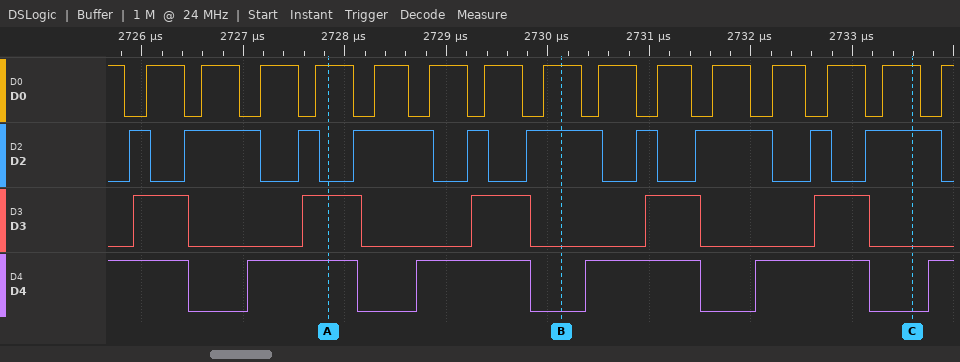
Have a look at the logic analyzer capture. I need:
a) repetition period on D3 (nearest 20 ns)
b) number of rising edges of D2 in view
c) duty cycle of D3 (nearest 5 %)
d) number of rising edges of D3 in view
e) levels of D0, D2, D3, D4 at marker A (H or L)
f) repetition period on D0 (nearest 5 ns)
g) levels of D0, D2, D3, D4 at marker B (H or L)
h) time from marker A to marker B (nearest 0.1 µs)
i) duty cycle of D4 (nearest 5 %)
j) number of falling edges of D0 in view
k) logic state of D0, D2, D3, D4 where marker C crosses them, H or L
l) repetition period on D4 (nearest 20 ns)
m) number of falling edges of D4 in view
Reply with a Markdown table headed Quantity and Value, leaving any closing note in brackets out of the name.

| Quantity | Value |
|---|---|
| repetition period on D3 | 1680 ns |
| number of rising edges of D2 in view | 10 |
| duty cycle of D3 | 35 % |
| number of rising edges of D3 in view | 5 |
| levels of D0, D2, D3, D4 at marker A | D0=H, D2=L, D3=H, D4=H |
| repetition period on D0 | 560 ns |
| levels of D0, D2, D3, D4 at marker B | D0=H, D2=H, D3=L, D4=L |
| time from marker A to marker B | 2.3 µs |
| duty cycle of D4 | 65 % |
| number of falling edges of D0 in view | 15 |
| logic state of D0, D2, D3, D4 where marker C crosses them, H or L | D0=H, D2=H, D3=L, D4=L |
| repetition period on D4 | 1680 ns |
| number of falling edges of D4 in view | 5 |
